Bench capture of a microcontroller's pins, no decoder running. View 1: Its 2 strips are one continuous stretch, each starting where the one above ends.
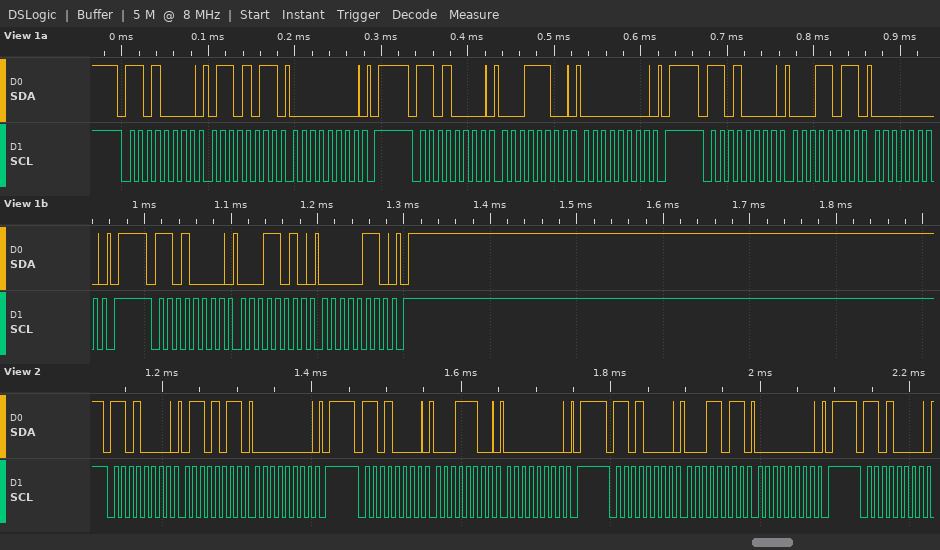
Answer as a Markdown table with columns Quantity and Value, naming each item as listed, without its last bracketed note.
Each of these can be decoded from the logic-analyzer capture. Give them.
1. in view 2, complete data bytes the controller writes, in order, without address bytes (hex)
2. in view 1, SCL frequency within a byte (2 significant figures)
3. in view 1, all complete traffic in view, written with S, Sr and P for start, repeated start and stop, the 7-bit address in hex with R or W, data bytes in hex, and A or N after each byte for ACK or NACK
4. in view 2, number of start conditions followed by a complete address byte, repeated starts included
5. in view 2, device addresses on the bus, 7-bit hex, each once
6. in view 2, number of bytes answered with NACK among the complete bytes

| Quantity | Value |
|---|---|
| in view 2, complete data bytes the controller writes, in order, without address bytes | 6B 00 1C 00 1B 00 |
| in view 1, SCL frequency within a byte | 100 kHz |
| in view 1, all complete traffic in view, written with S, Sr and P for start, repeated start and stop, the 7-bit address in hex with R or W, data bytes in hex, and A or N after each byte for ACK or NACK | S 68W A 6B A 00 A P S 68W A 1C A 00 A P S 68W A 1B A 00 A P S 68W A 1A A 06 A P |
| in view 2, number of start conditions followed by a complete address byte, repeated starts included | 4 |
| in view 2, device addresses on the bus, 7-bit hex, each once | 0x68 |
| in view 2, number of bytes answered with NACK among the complete bytes | 0 |
